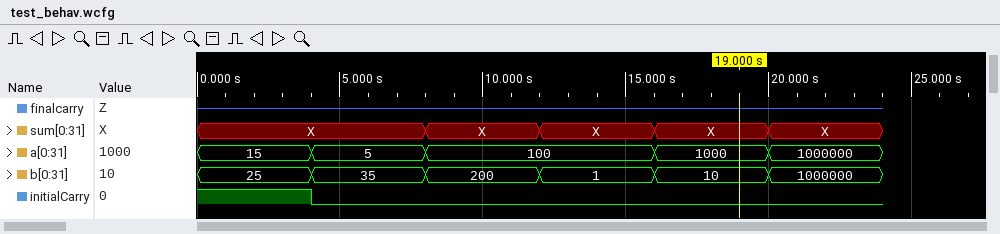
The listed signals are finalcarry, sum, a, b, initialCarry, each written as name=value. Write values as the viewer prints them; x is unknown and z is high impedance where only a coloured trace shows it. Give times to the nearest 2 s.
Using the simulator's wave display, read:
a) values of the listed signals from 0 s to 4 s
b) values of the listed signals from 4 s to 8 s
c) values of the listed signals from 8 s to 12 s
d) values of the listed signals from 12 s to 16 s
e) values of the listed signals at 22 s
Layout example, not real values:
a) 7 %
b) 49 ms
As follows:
a) finalcarry=z, sum=X, a=15, b=25, initialCarry=1
b) finalcarry=z, sum=X, a=5, b=35, initialCarry=0
c) finalcarry=z, sum=X, a=100, b=200, initialCarry=0
d) finalcarry=z, sum=X, a=100, b=1, initialCarry=0
e) finalcarry=z, sum=X, a=1000000, b=1000000, initialCarry=0
